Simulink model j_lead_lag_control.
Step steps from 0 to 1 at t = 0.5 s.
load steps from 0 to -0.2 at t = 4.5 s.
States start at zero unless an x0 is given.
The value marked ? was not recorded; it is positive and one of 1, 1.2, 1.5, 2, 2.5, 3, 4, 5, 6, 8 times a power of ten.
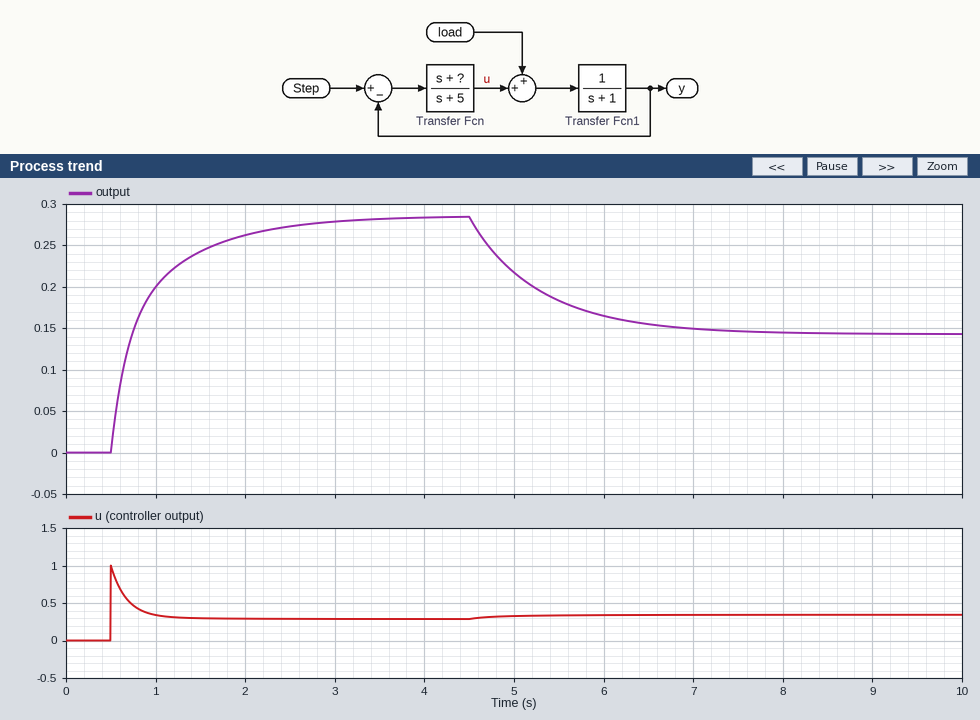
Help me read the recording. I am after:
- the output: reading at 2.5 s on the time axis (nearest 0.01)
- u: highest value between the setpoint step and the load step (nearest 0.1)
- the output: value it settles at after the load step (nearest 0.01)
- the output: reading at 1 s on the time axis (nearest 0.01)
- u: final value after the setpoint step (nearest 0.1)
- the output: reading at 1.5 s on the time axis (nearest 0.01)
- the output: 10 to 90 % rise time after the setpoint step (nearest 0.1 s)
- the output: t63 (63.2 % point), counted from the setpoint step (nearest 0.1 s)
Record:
0.27
1.0
0.14
0.20
0.3
0.24
1.3 s
0.4 s
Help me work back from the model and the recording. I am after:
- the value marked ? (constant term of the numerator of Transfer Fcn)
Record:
2
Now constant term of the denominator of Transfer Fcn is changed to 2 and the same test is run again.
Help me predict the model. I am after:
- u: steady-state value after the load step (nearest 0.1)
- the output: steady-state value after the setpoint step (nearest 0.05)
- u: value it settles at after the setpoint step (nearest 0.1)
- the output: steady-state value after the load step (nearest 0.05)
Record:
0.6
0.50
0.5
0.40
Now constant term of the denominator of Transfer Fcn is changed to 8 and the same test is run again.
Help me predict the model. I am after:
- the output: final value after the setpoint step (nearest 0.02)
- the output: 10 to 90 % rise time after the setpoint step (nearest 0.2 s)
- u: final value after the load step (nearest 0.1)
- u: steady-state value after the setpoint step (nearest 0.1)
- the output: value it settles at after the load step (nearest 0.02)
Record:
0.20
1.4 s
0.2
0.2
0.04
